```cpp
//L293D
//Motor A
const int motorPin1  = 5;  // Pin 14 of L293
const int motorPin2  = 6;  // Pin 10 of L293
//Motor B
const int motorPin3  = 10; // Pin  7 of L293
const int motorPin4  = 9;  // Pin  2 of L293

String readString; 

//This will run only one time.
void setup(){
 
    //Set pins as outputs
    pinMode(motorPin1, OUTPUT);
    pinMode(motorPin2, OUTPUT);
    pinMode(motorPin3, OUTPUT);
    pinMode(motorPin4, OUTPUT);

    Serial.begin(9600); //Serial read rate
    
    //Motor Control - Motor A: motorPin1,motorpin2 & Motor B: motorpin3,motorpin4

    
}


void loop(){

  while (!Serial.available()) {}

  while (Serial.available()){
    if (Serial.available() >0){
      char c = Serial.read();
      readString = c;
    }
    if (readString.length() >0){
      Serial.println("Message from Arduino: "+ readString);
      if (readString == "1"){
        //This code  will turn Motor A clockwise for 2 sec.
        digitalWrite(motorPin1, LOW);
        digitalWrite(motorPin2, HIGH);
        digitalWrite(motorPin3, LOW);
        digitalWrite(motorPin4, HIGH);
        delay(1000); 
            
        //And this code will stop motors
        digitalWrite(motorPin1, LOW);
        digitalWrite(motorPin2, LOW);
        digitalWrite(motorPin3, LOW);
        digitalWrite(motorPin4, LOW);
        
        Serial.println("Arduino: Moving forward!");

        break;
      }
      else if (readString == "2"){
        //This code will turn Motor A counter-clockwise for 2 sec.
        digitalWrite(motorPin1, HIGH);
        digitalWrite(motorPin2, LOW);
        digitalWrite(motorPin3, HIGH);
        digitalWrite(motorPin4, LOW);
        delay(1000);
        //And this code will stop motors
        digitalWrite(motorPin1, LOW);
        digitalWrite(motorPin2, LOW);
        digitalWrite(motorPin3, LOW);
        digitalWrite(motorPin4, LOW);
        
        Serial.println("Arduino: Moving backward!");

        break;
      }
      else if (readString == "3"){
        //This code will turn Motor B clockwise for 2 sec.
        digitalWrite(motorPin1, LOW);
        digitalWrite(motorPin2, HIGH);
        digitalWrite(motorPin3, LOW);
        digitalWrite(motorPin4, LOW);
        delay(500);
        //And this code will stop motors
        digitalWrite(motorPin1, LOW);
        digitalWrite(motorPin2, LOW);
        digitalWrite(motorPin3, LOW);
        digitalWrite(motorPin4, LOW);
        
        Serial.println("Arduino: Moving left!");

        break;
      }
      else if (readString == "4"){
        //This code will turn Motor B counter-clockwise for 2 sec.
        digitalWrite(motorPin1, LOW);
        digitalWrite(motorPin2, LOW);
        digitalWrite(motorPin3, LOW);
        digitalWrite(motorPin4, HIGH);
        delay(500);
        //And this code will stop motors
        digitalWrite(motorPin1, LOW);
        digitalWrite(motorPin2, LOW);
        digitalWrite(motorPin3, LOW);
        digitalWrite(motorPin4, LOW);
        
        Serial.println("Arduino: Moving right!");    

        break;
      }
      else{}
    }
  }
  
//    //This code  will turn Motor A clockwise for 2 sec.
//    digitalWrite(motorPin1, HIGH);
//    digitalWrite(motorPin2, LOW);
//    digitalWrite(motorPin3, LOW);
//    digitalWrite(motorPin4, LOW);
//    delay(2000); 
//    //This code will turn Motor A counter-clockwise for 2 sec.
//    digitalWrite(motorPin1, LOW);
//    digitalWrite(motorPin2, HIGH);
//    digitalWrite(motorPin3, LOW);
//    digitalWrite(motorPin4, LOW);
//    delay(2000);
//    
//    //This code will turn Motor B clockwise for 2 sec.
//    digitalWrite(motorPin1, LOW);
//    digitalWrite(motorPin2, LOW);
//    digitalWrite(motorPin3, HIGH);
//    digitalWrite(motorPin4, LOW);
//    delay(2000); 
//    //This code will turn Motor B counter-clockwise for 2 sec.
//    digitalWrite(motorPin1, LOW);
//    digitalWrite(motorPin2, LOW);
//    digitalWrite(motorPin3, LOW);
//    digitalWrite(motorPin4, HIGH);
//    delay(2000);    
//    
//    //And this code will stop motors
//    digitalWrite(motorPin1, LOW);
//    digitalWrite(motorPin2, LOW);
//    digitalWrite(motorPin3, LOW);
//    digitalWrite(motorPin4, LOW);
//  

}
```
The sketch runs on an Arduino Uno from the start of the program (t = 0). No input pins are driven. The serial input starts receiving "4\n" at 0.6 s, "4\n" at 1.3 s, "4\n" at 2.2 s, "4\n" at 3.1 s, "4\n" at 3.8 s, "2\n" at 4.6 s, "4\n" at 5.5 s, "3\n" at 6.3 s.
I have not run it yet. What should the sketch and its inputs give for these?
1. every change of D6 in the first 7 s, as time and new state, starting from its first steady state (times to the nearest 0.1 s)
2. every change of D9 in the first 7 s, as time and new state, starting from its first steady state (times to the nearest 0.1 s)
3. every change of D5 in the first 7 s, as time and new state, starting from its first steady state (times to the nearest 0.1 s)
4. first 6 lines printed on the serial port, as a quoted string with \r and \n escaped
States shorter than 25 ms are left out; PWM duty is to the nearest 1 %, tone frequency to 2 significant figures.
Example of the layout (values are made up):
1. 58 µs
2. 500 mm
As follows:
1. 0 s low; 6.3 s high; 6.8 s low
2. 0 s low; 0.6 s high; 1.1 s low; 1.3 s high; 1.8 s low; 2.2 s high; 2.7 s low; 3.1 s high; 3.6 s low; 3.8 s high; 4.3 s low; 5.6 s high; 6.1 s low
3. 0 s low; 4.6 s high; 5.6 s low
4. "Message from Arduino: 4\r\nArduino: Moving right!\r\nMessage from Arduino: \n\r\nMessage from Arduino: 4\r\nArduino: Moving right!\r\n"
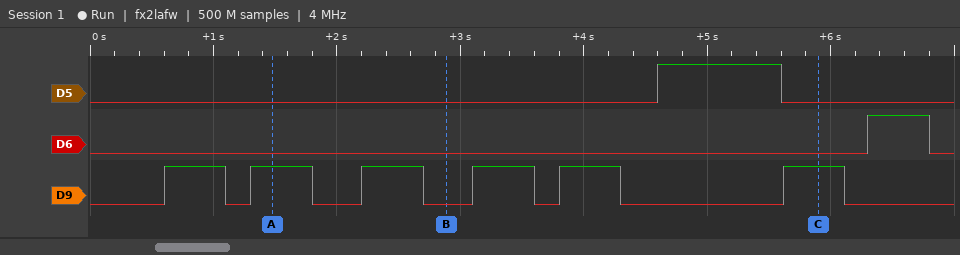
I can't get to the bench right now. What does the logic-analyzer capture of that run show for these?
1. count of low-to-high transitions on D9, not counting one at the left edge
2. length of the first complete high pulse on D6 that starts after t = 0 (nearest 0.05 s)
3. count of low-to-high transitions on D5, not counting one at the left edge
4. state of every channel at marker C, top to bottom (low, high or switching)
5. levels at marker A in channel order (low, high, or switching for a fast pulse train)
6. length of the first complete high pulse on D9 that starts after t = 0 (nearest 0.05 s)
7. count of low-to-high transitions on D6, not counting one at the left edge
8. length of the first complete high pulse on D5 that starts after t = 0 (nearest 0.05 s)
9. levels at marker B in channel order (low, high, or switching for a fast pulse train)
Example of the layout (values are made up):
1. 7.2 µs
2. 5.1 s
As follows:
1. 6
2. 0.50 s
3. 1
4. D5 low, D6 low, D9 high
5. D5 low, D6 low, D9 high
6. 0.50 s
7. 1
8. 1.00 s
9. D5 low, D6 low, D9 low
